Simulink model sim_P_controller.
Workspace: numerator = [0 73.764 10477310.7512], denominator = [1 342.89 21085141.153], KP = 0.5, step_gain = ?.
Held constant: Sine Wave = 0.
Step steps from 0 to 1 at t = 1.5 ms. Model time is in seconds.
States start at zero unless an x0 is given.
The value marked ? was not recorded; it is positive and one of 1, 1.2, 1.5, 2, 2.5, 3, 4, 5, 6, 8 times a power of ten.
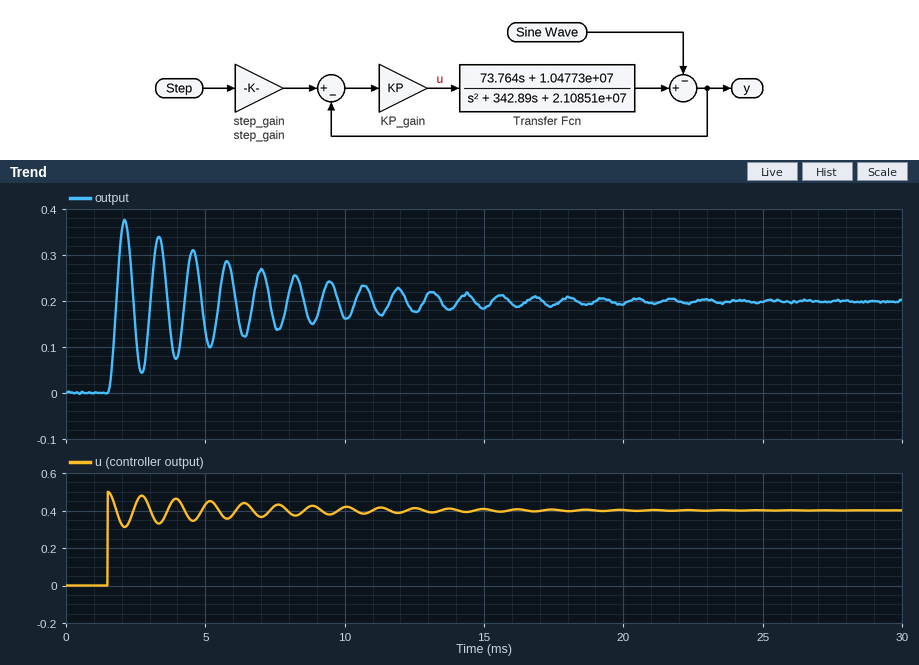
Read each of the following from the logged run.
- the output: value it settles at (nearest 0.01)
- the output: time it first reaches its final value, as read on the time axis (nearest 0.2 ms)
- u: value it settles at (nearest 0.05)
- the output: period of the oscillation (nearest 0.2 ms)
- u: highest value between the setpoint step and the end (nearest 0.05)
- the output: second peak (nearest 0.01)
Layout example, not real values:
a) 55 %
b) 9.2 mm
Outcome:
a) 0.20
b) 1.8 ms
c) 0.40
d) 1.2 ms
e) 0.50
f) 0.34
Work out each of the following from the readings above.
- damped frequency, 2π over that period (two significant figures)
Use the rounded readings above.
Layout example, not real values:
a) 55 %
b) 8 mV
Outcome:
a) 5.2 rad/ms
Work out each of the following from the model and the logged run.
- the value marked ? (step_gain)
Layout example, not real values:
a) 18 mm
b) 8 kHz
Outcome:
a) 1
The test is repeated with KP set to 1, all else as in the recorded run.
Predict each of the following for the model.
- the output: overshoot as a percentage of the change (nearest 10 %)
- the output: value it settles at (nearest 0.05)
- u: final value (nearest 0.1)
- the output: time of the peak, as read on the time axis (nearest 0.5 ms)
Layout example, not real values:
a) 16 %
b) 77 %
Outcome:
a) 90 %
b) 0.35
c) 0.7
d) 2.0 ms
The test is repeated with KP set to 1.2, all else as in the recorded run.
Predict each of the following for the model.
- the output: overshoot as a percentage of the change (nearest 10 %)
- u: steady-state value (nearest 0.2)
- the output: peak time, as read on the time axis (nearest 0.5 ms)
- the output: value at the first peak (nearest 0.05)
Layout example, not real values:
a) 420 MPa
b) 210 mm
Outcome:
a) 90 %
b) 0.8
c) 2.0 ms
d) 0.70
